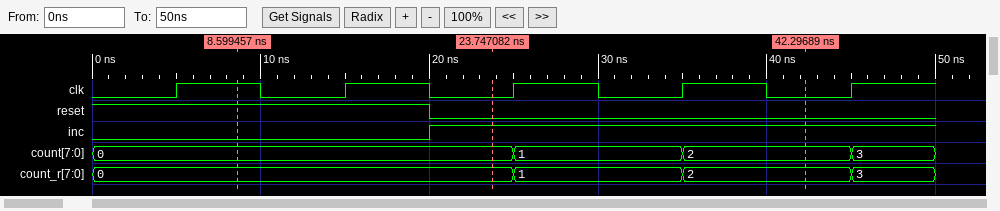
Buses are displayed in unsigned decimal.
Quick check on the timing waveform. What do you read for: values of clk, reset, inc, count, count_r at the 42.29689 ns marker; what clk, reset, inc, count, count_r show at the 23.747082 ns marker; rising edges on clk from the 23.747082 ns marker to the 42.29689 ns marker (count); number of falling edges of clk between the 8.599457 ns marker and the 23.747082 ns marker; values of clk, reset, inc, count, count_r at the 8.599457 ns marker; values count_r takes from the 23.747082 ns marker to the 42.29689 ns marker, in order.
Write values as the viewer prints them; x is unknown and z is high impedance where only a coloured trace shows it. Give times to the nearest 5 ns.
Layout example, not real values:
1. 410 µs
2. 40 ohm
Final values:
1. clk=0, reset=0, inc=1, count=2, count_r=2
2. clk=0, reset=0, inc=1, count=0, count_r=0
3. 2
4. 2
5. clk=1, reset=1, inc=0, count=0, count_r=0
6. 0, 1, 2
